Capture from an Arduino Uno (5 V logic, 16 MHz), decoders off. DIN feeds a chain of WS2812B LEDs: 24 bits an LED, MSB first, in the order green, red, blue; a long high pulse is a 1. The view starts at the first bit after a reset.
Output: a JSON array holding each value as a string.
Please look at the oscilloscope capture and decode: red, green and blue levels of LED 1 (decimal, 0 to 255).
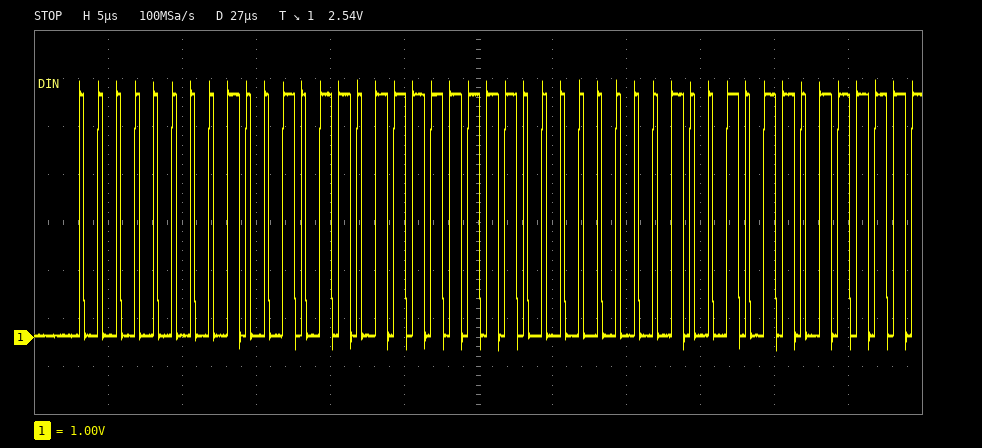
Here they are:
["150, 0, 255"]
